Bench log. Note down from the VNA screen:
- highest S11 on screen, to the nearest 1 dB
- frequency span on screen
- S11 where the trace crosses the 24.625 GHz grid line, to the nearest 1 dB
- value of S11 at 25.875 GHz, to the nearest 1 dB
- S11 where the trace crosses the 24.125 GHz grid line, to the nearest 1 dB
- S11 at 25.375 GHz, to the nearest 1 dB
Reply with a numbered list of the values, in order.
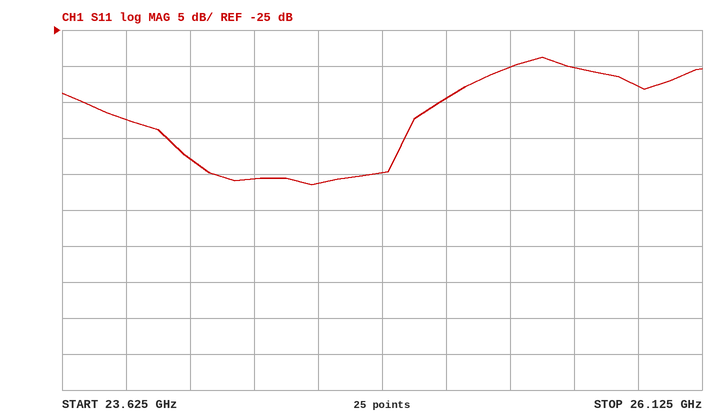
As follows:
1. -29 dB
2. 2.5 GHz
3. -46 dB
4. -33 dB
5. -43 dB
6. -30 dB
